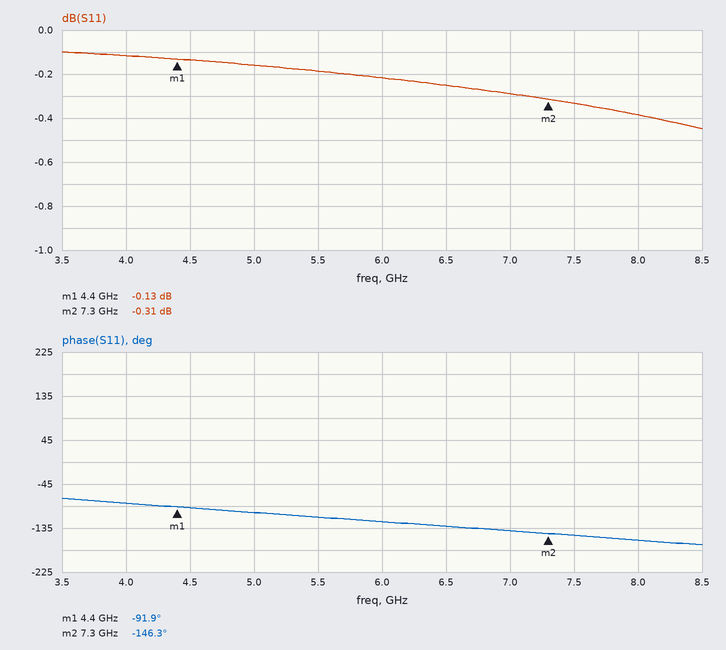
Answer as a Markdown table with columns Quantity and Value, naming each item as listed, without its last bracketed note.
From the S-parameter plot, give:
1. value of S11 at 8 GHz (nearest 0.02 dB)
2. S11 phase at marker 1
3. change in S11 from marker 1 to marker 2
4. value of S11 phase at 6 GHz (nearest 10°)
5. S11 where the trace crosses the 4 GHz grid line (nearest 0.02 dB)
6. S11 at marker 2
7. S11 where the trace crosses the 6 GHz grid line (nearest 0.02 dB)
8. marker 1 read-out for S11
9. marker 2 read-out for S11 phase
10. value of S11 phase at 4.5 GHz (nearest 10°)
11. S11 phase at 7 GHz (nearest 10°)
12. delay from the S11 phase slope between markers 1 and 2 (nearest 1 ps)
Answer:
| Quantity | Value |
|---|---|
| value of S11 at 8 GHz | -0.38 dB |
| S11 phase at marker 1 | -91.9° |
| change in S11 from marker 1 to marker 2 | -0.18 dB |
| value of S11 phase at 6 GHz | -120° |
| S11 where the trace crosses the 4 GHz grid line | -0.12 dB |
| S11 at marker 2 | -0.31 dB |
| S11 where the trace crosses the 6 GHz grid line | -0.22 dB |
| marker 1 read-out for S11 | -0.13 dB |
| marker 2 read-out for S11 phase | -146.3° |
| value of S11 phase at 4.5 GHz | -90° |
| S11 phase at 7 GHz | -140° |
| delay from the S11 phase slope between markers 1 and 2 | 52 ps |
